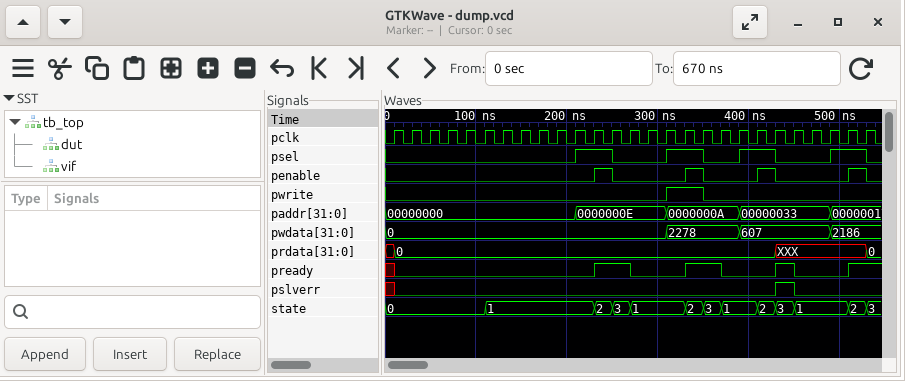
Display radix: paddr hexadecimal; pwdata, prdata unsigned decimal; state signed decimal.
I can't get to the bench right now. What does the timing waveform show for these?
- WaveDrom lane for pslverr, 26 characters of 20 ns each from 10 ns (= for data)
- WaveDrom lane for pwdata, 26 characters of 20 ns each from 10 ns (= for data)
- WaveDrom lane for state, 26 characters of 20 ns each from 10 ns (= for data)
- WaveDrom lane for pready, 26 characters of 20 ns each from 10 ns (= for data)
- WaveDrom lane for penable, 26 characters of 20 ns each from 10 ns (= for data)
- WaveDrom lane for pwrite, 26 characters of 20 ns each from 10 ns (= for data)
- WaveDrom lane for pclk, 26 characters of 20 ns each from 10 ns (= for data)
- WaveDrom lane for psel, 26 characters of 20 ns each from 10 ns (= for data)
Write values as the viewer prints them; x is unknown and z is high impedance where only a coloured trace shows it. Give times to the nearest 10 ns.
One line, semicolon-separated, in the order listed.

{name: 'pslverr', wave: '0....................10...'}; {name: 'pwdata', wave: '=..............=...=....=.', data: '0 2278 607 2186'}; {name: 'state', wave: '=....=.....===..===.===..=', data: '0 1 2 3 1 2 3 1 2 3 1 2'}; {name: 'pready', wave: '0..........1.0..1.0..10..1'}; {name: 'penable', wave: '0..........10...10..10...1'}; {name: 'pwrite', wave: '0..............1.0........'}; {name: 'pclk', wave: 'p.........................'}; {name: 'psel', wave: '0.........1.0..1.0.1.0..1.'}
